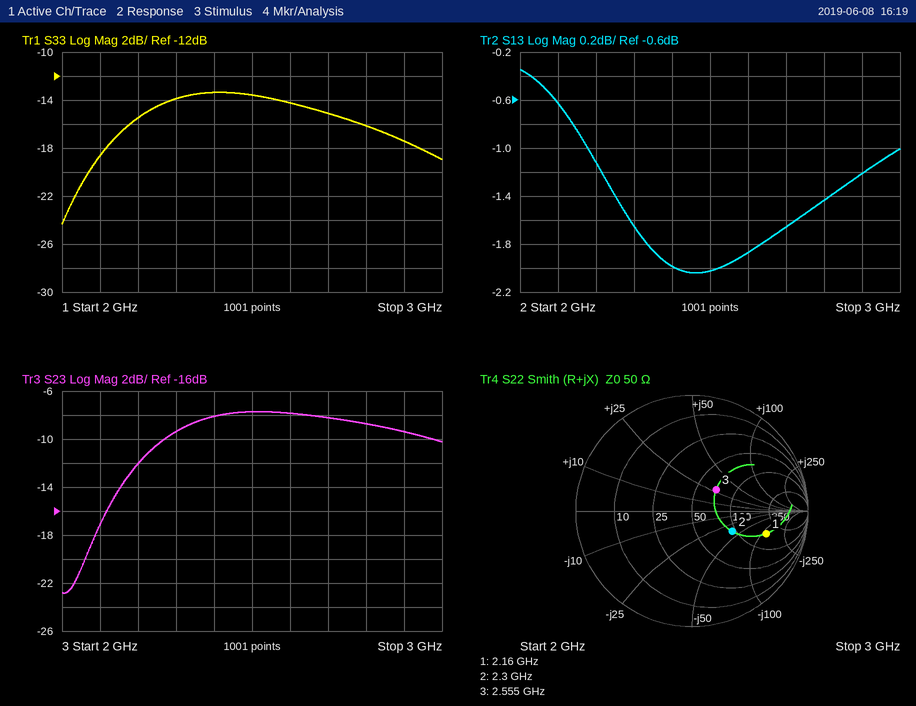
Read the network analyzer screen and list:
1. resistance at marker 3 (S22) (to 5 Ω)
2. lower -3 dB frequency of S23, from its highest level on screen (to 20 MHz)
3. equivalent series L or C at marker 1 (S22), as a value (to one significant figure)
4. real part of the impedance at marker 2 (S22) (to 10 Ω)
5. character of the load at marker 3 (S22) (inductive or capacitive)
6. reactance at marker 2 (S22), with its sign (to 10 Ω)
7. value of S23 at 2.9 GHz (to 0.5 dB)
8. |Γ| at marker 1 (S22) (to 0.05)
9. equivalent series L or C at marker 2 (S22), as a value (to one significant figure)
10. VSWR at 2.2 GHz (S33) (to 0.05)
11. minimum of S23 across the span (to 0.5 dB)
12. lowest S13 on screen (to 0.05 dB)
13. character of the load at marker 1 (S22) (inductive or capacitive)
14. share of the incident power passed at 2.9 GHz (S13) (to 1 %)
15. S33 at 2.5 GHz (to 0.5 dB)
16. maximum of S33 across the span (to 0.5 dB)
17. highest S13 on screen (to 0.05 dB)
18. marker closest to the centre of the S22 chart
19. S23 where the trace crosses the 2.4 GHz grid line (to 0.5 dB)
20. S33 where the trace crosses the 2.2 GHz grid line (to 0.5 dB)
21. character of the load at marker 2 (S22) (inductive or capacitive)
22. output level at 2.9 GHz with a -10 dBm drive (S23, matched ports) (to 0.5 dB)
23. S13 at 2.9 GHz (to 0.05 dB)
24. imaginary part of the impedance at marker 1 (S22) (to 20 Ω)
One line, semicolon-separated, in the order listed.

70 Ω; 2.24 GHz; 600 fF; 90 Ω; inductive; -40 Ω; -9.5 dB; 0.65; 2 pF; 1.40; -23.0 dB; -2.05 dB; capacitive; 76 %; -13.5 dB; -13.5 dB; -0.35 dB; marker 3; -8.0 dB; -15.5 dB; capacitive; -19.5 dBm; -1.20 dB; -120 Ω
